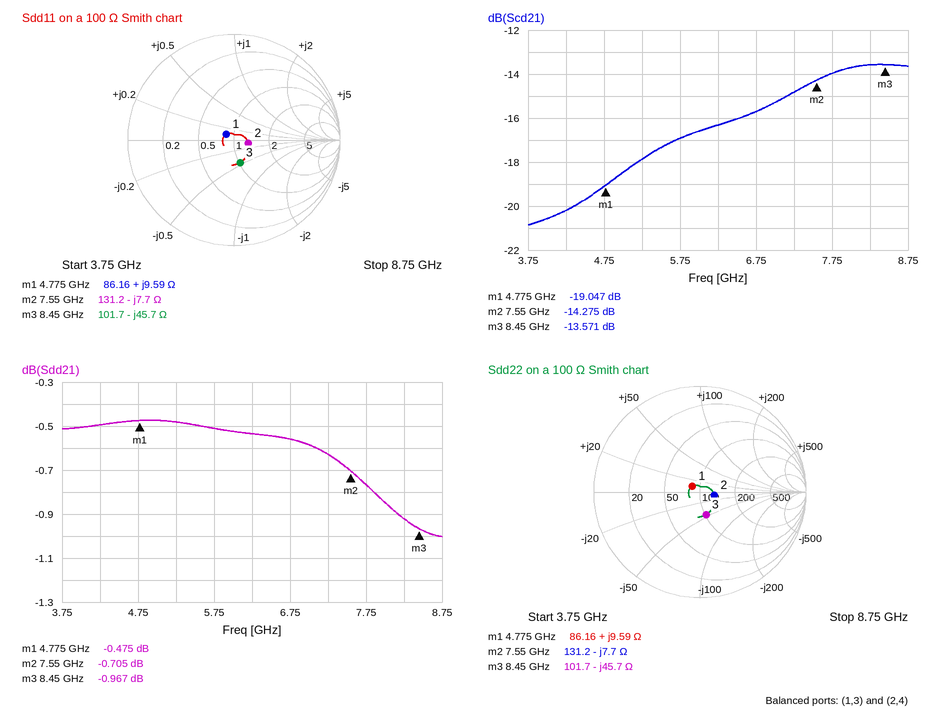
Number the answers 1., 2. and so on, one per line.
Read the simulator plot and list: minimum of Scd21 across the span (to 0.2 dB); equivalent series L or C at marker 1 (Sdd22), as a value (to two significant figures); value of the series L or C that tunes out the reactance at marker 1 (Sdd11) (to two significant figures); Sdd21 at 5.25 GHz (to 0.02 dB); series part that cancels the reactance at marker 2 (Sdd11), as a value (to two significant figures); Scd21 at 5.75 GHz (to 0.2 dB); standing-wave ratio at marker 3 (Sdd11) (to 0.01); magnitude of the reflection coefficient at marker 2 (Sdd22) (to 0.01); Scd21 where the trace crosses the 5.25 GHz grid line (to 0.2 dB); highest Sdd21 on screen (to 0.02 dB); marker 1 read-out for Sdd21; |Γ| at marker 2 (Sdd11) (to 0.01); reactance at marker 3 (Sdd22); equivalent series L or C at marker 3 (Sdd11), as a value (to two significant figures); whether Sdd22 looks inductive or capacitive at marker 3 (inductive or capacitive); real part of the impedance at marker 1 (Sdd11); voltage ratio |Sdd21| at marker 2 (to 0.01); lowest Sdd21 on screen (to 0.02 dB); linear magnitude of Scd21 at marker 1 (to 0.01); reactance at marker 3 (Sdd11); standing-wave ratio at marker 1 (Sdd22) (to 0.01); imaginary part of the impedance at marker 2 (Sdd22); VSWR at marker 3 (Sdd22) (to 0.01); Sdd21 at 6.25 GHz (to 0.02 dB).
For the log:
1. -20.8 dB
2. 320 pH
3. 3.5 pF
4. -0.48 dB
5. 160 pH
6. -17.0 dB
7. 1.57
8. 0.14
9. -17.8 dB
10. -0.48 dB
11. -0.475 dB
12. 0.14
13. -45.7 Ω
14. 410 fF
15. capacitive
16. 86.16 Ω
17. 0.92
18. -1.00 dB
19. 0.11
20. -45.7 Ω
21. 1.20
22. -7.7 Ω
23. 1.57
24. -0.54 dB
